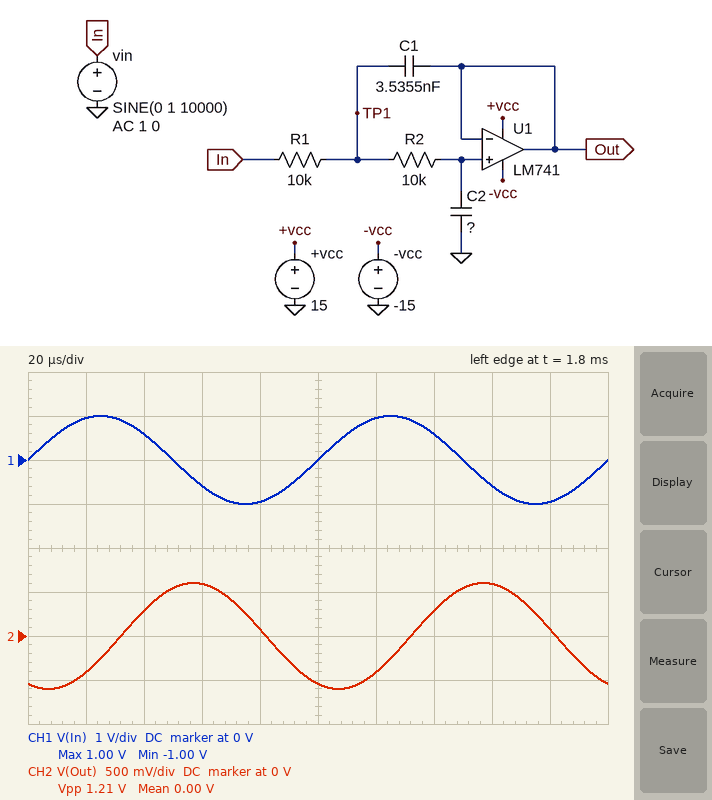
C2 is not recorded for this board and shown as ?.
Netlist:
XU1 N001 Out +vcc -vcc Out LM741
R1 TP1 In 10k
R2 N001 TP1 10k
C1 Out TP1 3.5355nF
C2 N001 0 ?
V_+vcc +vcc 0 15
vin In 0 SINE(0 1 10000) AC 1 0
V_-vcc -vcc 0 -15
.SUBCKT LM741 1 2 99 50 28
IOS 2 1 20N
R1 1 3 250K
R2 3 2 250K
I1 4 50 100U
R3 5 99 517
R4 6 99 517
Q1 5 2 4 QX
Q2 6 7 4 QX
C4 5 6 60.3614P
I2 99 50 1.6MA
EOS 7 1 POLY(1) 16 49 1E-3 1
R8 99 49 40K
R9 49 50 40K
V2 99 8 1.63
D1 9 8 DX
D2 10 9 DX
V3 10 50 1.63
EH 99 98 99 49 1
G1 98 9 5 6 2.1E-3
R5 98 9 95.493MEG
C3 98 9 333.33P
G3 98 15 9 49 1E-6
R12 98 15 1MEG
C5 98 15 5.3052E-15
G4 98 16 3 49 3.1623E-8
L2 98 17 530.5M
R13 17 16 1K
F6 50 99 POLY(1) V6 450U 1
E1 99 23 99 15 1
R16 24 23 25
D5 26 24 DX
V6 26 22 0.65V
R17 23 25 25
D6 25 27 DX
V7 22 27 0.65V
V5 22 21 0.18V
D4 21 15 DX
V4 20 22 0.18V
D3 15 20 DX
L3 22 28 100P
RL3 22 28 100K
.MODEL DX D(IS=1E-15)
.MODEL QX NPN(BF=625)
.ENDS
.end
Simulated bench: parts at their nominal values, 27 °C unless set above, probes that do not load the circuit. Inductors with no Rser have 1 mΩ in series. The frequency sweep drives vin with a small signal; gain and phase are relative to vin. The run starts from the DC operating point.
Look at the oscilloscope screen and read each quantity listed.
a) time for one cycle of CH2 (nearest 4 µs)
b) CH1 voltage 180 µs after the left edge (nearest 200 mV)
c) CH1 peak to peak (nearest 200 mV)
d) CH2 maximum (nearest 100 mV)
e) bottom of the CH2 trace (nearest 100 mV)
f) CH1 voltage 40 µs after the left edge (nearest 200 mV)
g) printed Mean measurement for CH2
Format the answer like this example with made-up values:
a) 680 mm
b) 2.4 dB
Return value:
a) 100 µs
b) -1.0 V
c) 2.0 V
d) 600 mV
e) -600 mV
f) 600 mV
g) 0.00 V
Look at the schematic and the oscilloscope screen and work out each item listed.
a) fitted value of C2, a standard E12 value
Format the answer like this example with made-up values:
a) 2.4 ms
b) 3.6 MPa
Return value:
a) 1.2 nF
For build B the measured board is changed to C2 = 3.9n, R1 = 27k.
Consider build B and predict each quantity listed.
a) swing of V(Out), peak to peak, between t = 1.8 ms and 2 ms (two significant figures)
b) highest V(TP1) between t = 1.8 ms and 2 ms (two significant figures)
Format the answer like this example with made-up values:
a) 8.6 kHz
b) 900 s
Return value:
a) 120 mV
b) 160 mV
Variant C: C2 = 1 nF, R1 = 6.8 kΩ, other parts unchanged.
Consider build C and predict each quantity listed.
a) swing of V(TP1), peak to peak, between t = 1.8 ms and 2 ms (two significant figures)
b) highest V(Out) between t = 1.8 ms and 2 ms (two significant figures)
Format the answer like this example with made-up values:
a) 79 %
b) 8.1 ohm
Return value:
a) 2.2 V
b) 950 mV
